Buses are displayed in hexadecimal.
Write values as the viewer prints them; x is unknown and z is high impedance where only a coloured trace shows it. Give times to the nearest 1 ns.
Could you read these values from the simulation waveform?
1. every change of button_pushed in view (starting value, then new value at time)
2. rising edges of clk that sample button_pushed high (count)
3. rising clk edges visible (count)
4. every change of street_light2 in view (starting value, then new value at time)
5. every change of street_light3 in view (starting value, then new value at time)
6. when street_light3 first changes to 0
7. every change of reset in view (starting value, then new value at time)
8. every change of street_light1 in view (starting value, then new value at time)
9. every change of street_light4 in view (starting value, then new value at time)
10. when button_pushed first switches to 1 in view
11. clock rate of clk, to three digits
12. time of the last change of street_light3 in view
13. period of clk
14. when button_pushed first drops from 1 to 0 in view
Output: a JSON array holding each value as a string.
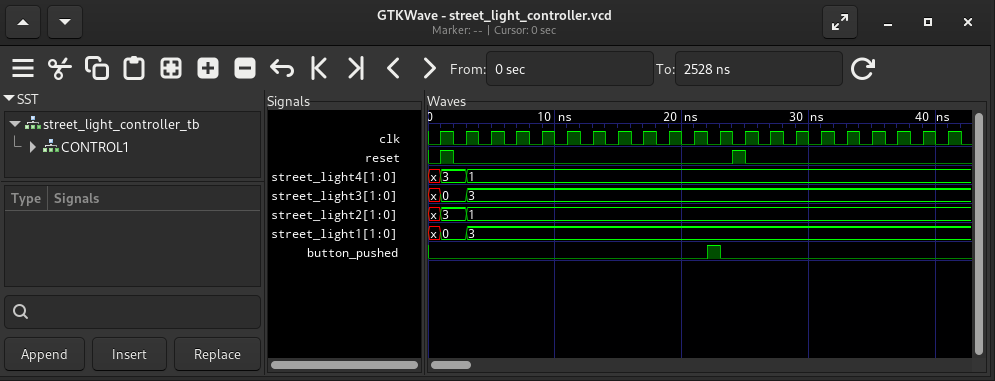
["0, 1 at 22 ns, 0 at 23 ns", "1", "21", "x, 3 at 1 ns, 1 at 3 ns", "x, 0 at 1 ns, 3 at 3 ns", "1 ns", "0, 1 at 1 ns, 0 at 2 ns, 1 at 24 ns, 0 at 25 ns", "x, 0 at 1 ns, 3 at 3 ns", "x, 3 at 1 ns, 1 at 3 ns", "22 ns", "500 MHz", "3 ns", "2 ns", "23 ns"]
